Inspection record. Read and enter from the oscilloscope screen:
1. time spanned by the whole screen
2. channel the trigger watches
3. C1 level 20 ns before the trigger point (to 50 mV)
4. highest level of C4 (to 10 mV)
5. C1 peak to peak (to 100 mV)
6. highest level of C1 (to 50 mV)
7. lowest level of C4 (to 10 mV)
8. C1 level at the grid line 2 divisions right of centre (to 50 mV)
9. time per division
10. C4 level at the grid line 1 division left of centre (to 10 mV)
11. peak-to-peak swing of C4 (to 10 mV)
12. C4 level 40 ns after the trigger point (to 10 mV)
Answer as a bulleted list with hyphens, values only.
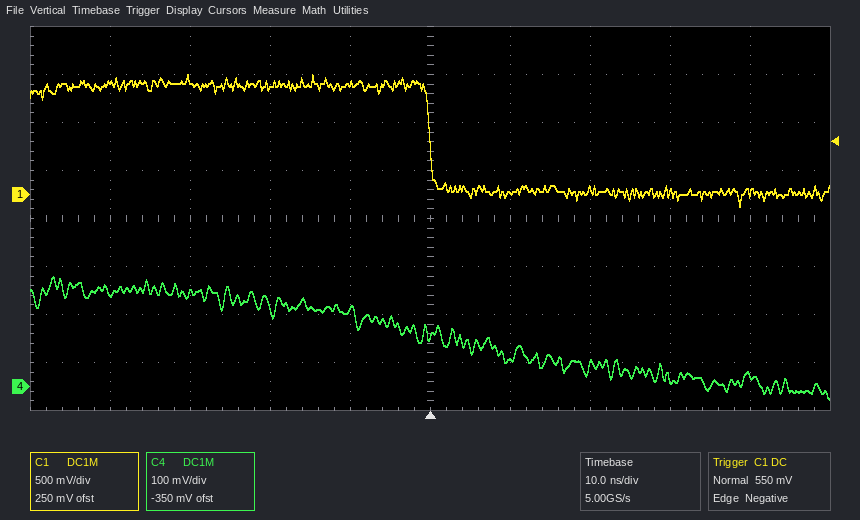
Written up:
- 100 ns
- C1
- 1.15 V
- 230 mV
- 1.40 V
- 1.25 V
- -30 mV
- 50 mV
- 10 ns
- 160 mV
- 260 mV
- 20 mV
